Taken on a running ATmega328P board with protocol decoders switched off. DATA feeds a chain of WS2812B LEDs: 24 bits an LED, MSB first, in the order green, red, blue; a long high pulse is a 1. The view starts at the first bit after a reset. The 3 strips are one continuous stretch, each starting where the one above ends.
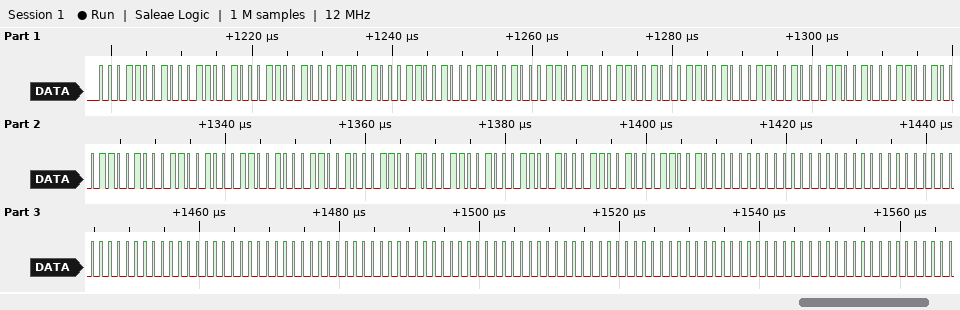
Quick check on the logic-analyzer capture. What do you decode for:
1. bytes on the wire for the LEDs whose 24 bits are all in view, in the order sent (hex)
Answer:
19 19 19 19 19 19 19 19 19 19 19 19 19 19 19 19 19 19 19 19 19 00 00 00 00 00 00 00 00 00 00 00 00 00 00 00
